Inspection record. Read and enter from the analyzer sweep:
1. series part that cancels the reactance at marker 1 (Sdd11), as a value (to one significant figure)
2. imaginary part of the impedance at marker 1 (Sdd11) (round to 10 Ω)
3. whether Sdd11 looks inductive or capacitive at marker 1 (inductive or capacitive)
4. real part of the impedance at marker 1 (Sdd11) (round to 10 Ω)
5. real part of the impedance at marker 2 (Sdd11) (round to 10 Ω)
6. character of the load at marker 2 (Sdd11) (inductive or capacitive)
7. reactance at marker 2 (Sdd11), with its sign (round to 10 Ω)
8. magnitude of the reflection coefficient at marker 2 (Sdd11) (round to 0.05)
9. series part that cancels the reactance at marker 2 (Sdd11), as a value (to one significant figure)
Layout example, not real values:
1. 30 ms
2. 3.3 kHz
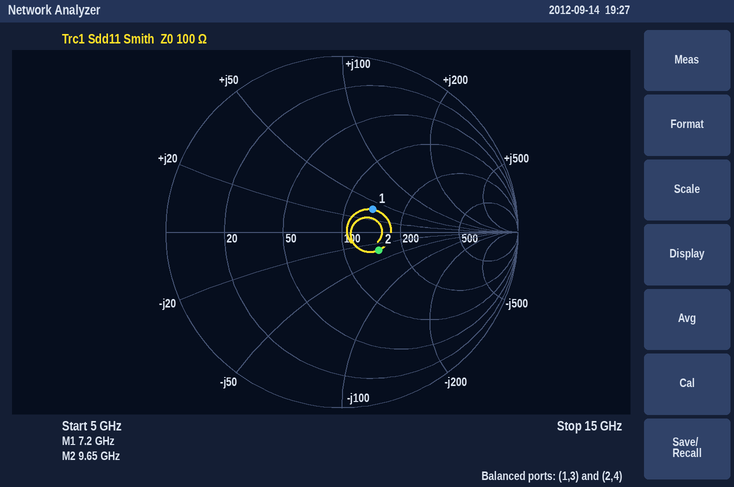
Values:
1. 600 fF
2. +40 Ω
3. inductive
4. 140 Ω
5. 150 Ω
6. capacitive
7. -30 Ω
8. 0.25
9. 500 pH
